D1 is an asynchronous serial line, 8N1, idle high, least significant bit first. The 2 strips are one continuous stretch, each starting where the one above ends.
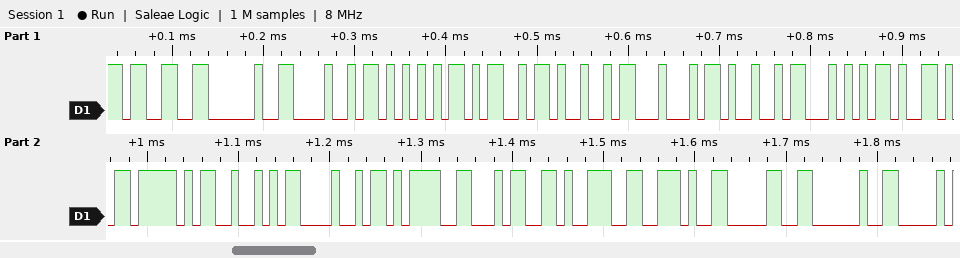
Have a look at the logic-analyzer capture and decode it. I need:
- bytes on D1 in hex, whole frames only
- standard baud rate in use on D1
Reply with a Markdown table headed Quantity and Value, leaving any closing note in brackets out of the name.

| Quantity | Value |
|---|---|
| bytes on D1 in hex, whole frames only | 0x33 0x20 0x48 0x55 0x4D 0x49 0x44 0x49 0x54 0x59 0x5F 0x52 0x48 0x3D 0x34 0x39 0x2E 0x30 0x20 |
| standard baud rate in use on D1 | 115200 baud |
